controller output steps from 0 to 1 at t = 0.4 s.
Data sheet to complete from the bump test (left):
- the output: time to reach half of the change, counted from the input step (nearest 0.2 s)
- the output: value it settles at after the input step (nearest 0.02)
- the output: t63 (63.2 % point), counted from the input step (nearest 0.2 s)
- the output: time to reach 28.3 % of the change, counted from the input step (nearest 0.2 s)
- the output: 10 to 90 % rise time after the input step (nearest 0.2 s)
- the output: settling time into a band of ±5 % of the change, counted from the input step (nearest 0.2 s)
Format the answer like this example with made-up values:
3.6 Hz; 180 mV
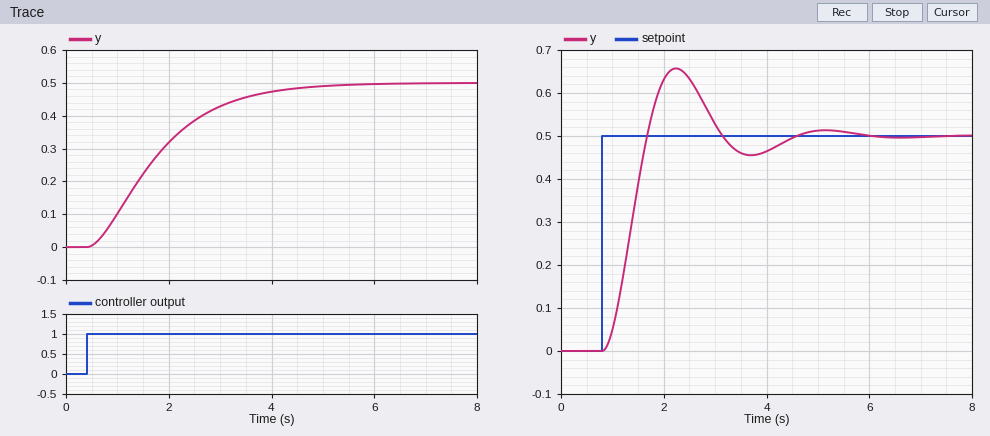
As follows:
1.2 s; 0.50; 1.6 s; 0.8 s; 2.6 s; 3.6 s
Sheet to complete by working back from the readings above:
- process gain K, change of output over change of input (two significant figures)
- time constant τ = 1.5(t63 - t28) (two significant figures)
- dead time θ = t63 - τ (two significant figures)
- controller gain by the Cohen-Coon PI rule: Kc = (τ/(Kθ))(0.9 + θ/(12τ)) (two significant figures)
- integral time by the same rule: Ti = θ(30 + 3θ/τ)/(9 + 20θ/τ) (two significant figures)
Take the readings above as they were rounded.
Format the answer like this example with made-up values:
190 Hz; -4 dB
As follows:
0.50; 1.2 s; 0.40 s; 5.6; 0.79 s
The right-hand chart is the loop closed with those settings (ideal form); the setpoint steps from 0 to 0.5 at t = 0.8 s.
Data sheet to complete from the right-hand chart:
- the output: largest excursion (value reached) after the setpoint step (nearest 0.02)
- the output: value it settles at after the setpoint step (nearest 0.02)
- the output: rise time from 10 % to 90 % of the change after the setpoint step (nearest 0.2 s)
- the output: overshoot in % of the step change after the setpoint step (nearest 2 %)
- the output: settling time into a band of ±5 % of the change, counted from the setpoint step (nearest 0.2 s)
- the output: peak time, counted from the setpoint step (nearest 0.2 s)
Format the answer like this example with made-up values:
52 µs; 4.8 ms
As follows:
0.66; 0.50; 0.6 s; 32 %; 3.4 s; 1.4 s
